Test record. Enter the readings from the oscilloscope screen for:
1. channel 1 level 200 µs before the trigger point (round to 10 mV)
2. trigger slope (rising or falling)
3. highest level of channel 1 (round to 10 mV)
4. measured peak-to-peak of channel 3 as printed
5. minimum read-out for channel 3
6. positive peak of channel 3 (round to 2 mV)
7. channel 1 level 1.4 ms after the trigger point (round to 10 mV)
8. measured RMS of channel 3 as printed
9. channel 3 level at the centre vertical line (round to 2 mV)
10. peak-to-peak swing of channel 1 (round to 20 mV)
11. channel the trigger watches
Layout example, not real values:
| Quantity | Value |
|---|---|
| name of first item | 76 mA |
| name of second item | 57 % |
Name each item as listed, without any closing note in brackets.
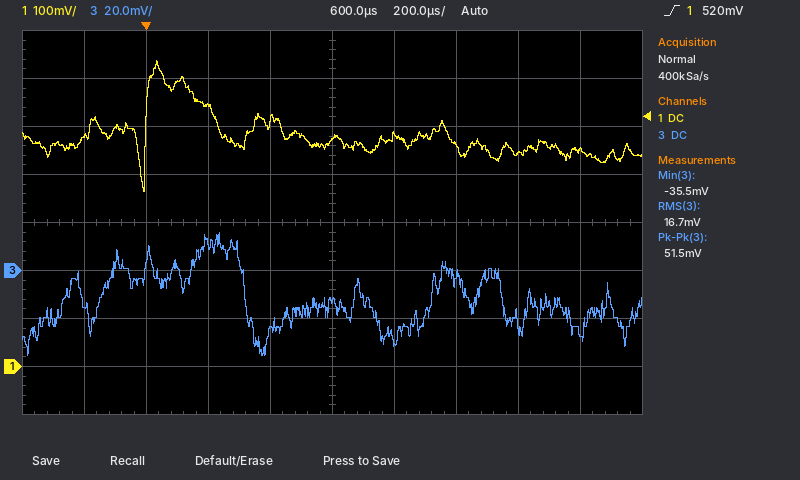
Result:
| Quantity | Value |
|---|---|
| channel 1 level 200 µs before the trigger point | 480 mV |
| trigger slope | rising |
| highest level of channel 1 | 640 mV |
| measured peak-to-peak of channel 3 as printed | 51.5 mV |
| minimum read-out for channel 3 | -35.5 mV |
| positive peak of channel 3 | 16 mV |
| channel 1 level 1.4 ms after the trigger point | 450 mV |
| measured RMS of channel 3 as printed | 16.7 mV |
| channel 3 level at the centre vertical line | -12 mV |
| peak-to-peak swing of channel 1 | 280 mV |
| channel the trigger watches | channel 1 |
